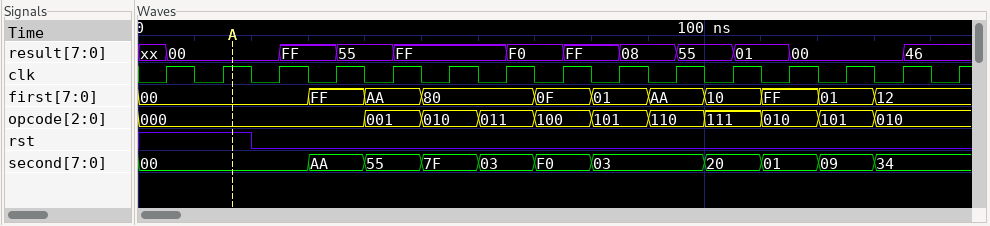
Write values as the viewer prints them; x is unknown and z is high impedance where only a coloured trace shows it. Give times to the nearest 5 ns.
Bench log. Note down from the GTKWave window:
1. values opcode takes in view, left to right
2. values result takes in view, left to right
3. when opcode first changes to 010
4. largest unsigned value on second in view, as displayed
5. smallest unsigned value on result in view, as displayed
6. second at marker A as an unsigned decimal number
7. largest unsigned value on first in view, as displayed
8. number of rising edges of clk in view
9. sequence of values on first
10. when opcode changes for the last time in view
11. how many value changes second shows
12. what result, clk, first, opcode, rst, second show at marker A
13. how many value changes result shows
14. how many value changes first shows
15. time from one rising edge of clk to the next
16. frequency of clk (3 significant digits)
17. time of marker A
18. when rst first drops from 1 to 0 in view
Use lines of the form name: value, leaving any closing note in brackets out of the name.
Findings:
values opcode takes in view, left to right: 000, 001, 010, 011, 100, 101, 110, 111, 010, 101, 010
values result takes in view, left to right: xx, 00, FF, 55, FF, F0, FF, 08, 55, 01, 00, 46
when opcode first changes to 010: 50 ns
largest unsigned value on second in view, as displayed: F0
smallest unsigned value on result in view, as displayed: 00
second at marker A as an unsigned decimal number: 0
largest unsigned value on first in view, as displayed: FF
number of rising edges of clk in view: 15
sequence of values on first: 00, FF, AA, 80, 0F, 01, AA, 10, FF, 01, 12
when opcode changes for the last time in view: 130 ns
how many value changes second shows: 10
what result, clk, first, opcode, rst, second show at marker A: result=00, clk=1, first=00, opcode=000, rst=1, second=00
how many value changes result shows: 11
how many value changes first shows: 10
time from one rising edge of clk to the next: 10 ns
frequency of clk: 100 MHz
time of marker A: 15 ns
when rst first drops from 1 to 0 in view: 20 ns
